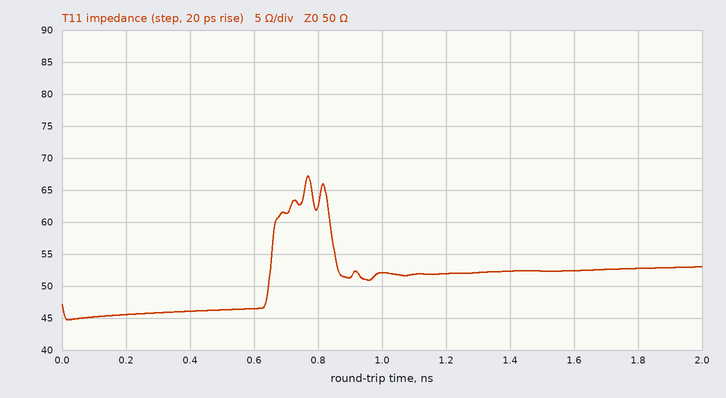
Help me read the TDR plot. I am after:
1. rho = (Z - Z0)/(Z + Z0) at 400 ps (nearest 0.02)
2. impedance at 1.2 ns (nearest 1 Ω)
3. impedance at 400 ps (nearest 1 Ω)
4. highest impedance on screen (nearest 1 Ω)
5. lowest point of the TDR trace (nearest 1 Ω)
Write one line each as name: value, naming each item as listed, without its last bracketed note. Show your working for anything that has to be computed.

rho = (Z - Z0)/(Z + Z0) at 400 ps: (46 − 50)/(46 + 50) ≈ -0.04
impedance at 1.2 ns: 52 Ω
impedance at 400 ps: 46 Ω
highest impedance on screen: 67 Ω
lowest point of the TDR trace: 45 Ω
